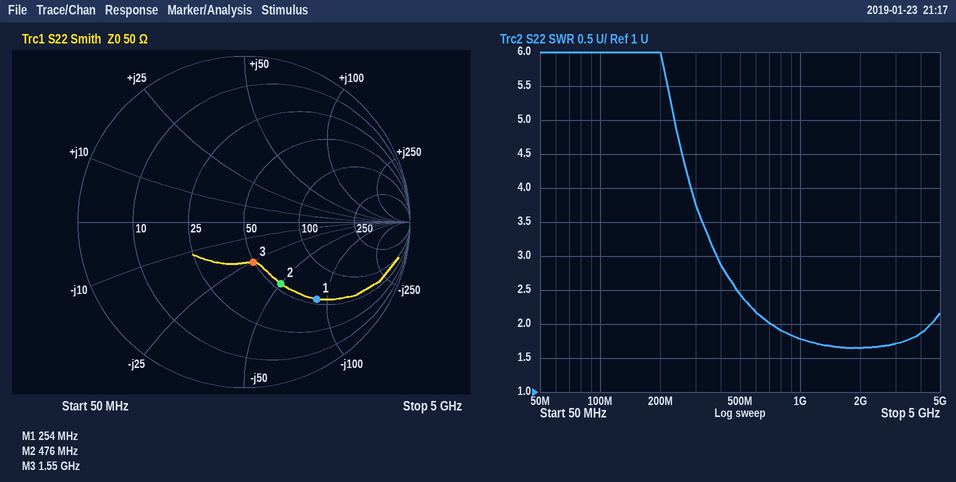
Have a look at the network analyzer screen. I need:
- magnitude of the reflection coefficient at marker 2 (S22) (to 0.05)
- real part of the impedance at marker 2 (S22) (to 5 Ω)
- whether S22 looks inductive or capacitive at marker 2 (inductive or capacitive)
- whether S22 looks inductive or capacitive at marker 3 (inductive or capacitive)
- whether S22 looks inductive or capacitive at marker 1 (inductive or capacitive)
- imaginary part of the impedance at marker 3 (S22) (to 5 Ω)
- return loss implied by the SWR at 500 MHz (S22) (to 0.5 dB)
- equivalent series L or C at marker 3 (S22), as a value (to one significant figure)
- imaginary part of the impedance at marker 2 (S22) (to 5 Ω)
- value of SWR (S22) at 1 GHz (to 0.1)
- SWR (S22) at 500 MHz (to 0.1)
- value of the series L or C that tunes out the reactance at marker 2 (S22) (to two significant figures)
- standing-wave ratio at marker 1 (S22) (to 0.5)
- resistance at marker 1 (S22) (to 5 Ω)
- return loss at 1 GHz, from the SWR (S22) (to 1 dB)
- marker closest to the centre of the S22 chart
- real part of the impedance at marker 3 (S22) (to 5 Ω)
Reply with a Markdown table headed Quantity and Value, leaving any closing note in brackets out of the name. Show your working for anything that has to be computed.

| Quantity | Value |
|---|---|
| magnitude of the reflection coefficient at marker 2 (S22) | 0.45 |
| real part of the impedance at marker 2 (S22) | 55 Ω |
| whether S22 looks inductive or capacitive at marker 2 | capacitive |
| whether S22 looks inductive or capacitive at marker 3 | capacitive |
| whether S22 looks inductive or capacitive at marker 1 | capacitive |
| imaginary part of the impedance at marker 3 (S22) | -25 Ω |
| return loss implied by the SWR at 500 MHz (S22) | −20 log10((2.4 − 1)/(2.4 + 1)) ≈ 7.71 dB, so 7.5 dB to the nearest 0.5 dB |
| equivalent series L or C at marker 3 (S22), as a value | C = 1/(2π × 1.55 GHz × 25 Ω) ≈ 4 pF |
| imaginary part of the impedance at marker 2 (S22) | -50 Ω |
| value of SWR (S22) at 1 GHz | 1.8 |
| SWR (S22) at 500 MHz | 2.4 |
| value of the series L or C that tunes out the reactance at marker 2 (S22) | L = 50 Ω/(2π × 476 MHz) ≈ 17 nH |
| standing-wave ratio at marker 1 (S22) | 4.5 |
| resistance at marker 1 (S22) | 55 Ω |
| return loss at 1 GHz, from the SWR (S22) | −20 log10((1.8 − 1)/(1.8 + 1)) ≈ 11 dB |
| marker closest to the centre of the S22 chart | marker 3 |
| real part of the impedance at marker 3 (S22) | 50 Ω |
